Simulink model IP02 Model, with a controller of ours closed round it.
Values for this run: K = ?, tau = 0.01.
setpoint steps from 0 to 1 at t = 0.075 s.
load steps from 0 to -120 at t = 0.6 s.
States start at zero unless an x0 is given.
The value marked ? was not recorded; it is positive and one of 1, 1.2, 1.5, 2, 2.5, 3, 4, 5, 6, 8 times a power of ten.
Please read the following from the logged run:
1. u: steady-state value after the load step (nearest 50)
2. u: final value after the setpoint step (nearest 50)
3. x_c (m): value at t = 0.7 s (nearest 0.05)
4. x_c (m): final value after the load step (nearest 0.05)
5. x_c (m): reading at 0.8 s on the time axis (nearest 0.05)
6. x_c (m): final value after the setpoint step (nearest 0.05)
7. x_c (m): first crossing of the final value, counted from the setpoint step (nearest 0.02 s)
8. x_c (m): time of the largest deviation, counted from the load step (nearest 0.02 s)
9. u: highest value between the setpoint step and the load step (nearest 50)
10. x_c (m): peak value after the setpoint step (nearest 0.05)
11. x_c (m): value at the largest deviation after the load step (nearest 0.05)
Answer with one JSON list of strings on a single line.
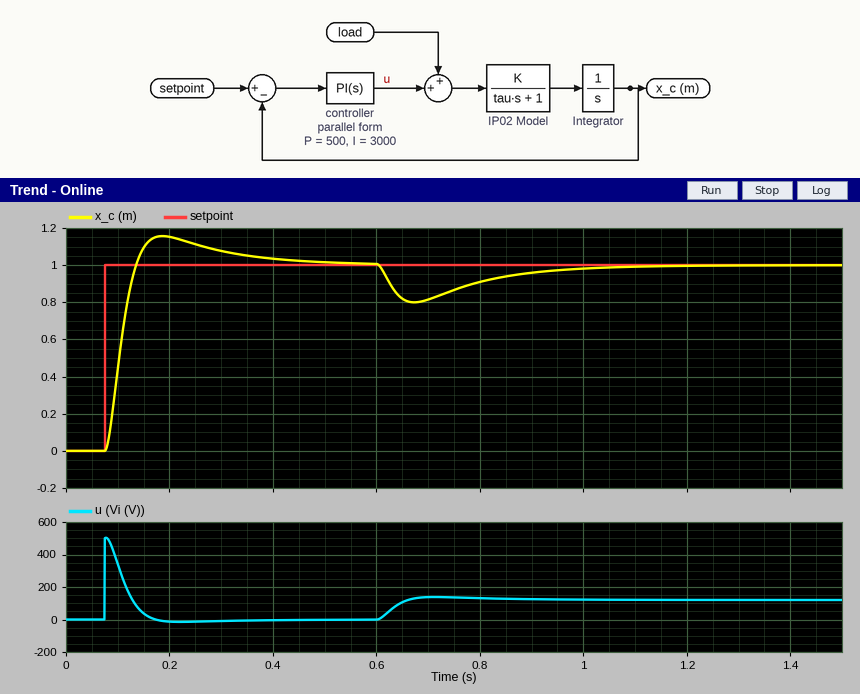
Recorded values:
["100", "0", "0.80", "1.00", "0.90", "1.00", "0.06 s", "0.08 s", "500", "1.15", "0.80"]
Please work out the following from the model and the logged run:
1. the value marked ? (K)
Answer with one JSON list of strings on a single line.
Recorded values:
["0.06"]
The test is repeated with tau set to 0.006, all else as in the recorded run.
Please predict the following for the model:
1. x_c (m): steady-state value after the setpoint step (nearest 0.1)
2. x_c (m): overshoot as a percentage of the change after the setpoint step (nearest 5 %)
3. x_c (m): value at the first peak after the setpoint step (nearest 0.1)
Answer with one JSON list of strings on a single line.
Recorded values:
["1.0", "15 %", "1.1"]
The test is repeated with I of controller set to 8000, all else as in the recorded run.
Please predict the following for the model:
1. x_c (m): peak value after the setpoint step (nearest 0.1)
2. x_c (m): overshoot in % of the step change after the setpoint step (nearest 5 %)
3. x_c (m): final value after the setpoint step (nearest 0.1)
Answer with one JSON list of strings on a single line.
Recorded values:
["1.3", "35 %", "1.0"]
